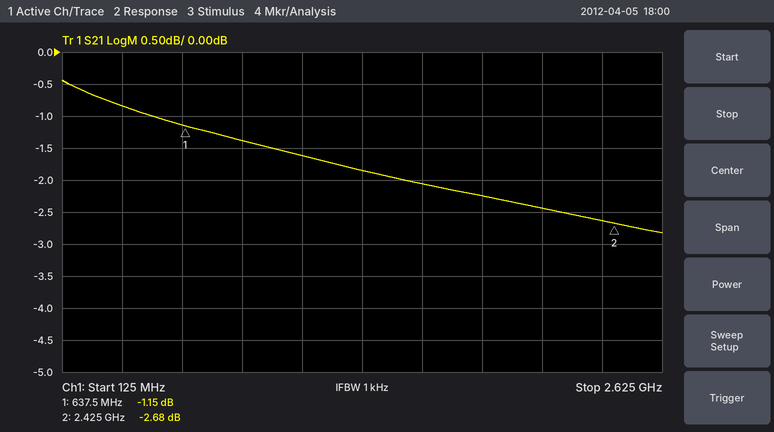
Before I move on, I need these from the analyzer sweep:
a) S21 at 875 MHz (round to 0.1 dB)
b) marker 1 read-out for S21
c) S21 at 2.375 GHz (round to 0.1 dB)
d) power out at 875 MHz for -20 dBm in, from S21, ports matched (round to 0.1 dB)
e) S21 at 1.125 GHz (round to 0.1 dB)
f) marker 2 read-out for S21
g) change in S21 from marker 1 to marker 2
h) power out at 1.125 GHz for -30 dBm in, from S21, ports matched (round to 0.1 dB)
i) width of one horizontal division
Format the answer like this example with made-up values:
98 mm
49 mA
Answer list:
-1.4 dB
-1.15 dB
-2.6 dB
-21.4 dBm
-1.6 dB
-2.68 dB
-1.53 dB
-31.6 dBm
250 MHz
